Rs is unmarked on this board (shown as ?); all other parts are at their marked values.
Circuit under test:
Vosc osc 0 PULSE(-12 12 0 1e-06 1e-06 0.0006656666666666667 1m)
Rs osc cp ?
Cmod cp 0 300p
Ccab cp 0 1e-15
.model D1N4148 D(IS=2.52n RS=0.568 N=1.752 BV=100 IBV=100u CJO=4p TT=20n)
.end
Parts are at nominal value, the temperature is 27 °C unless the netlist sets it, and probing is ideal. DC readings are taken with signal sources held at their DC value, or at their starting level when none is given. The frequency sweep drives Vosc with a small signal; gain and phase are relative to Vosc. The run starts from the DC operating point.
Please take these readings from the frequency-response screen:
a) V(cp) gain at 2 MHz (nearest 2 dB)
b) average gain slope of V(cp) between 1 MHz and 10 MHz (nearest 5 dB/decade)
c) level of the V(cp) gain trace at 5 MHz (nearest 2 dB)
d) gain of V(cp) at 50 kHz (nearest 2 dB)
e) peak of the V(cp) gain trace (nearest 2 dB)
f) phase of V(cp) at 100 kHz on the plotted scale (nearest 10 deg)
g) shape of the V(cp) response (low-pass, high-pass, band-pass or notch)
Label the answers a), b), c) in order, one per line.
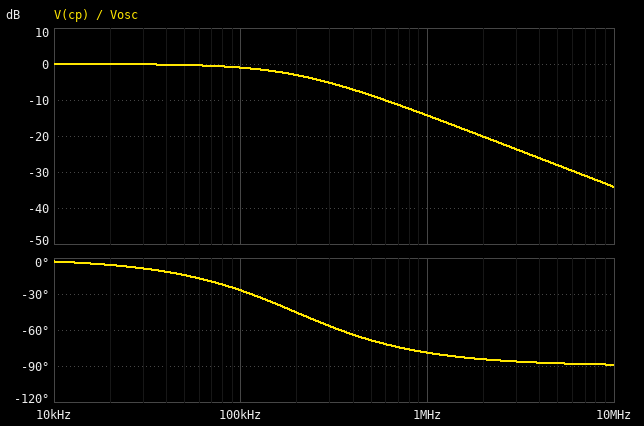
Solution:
a) -20 dB
b) -20 dB/decade
c) -28 dB
d) 0 dB
e) 0 dB
f) -30 deg
g) low-pass
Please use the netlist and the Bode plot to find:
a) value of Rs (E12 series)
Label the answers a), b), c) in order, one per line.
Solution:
a) 2.7 kΩ
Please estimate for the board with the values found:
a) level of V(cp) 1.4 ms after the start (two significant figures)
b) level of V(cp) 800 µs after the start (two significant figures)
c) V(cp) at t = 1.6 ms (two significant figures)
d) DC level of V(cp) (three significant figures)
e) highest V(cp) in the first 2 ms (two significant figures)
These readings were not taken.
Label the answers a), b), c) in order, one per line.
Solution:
a) 12 V
b) -12 V
c) 12 V
d) -12.0 V
e) 12 V
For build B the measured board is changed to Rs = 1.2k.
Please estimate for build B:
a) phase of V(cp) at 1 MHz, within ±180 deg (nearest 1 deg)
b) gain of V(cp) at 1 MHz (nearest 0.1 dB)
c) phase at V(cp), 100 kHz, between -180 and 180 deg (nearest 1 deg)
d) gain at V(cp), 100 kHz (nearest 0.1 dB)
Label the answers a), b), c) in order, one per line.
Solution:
a) -66 deg
b) -7.9 dB
c) -13 deg
d) -0.2 dB
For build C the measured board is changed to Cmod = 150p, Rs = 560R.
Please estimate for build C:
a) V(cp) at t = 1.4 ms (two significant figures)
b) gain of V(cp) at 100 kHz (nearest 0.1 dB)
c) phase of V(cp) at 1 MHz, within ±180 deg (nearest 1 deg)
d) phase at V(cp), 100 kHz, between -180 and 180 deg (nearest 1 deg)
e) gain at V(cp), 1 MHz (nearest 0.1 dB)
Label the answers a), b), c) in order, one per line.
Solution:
a) 12 V
b) 0 dB
c) -28 deg
d) -3 deg
e) -1.1 dB
